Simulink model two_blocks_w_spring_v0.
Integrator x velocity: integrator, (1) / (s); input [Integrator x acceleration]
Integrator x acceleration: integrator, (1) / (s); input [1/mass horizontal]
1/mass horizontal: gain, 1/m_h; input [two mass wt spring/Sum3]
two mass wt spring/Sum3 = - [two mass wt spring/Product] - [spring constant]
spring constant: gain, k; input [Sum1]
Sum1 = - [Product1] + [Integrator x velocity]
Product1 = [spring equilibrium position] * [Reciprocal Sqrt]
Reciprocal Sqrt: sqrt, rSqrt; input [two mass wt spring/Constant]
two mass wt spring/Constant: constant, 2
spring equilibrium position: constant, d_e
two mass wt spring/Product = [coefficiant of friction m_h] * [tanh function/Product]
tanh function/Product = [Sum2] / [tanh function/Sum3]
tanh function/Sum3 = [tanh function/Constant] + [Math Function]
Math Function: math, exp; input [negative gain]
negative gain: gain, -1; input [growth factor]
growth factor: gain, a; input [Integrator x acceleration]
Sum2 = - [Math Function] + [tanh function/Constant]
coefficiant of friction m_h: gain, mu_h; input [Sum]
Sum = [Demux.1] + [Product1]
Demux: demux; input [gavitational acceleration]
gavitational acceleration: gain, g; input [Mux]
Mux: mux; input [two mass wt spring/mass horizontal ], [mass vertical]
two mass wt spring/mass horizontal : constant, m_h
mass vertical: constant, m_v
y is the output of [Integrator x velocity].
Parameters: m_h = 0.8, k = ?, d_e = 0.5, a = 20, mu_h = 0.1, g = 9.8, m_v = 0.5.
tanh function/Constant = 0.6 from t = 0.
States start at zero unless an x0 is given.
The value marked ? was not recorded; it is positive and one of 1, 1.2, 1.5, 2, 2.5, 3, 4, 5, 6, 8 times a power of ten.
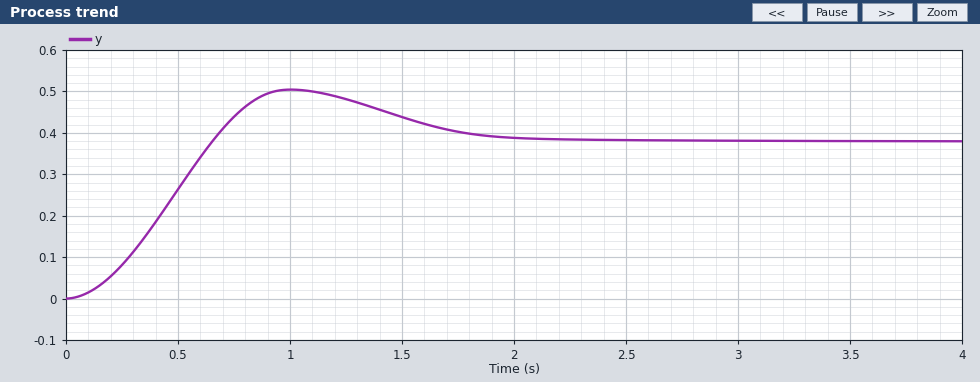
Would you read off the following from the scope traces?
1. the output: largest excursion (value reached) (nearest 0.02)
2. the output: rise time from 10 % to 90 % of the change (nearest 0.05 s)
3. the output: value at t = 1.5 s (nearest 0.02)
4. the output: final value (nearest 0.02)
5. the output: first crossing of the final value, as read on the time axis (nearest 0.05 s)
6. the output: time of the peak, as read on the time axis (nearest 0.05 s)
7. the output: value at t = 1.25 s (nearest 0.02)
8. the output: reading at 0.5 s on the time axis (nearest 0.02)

0.50
0.45 s
0.44
0.38
0.65 s
1.00 s
0.48
0.26
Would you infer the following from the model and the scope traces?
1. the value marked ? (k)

8
